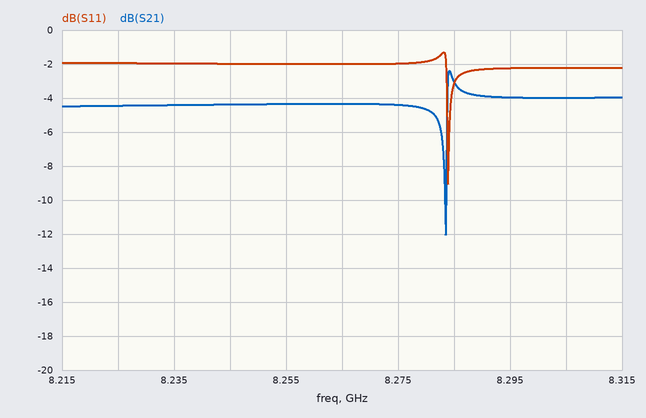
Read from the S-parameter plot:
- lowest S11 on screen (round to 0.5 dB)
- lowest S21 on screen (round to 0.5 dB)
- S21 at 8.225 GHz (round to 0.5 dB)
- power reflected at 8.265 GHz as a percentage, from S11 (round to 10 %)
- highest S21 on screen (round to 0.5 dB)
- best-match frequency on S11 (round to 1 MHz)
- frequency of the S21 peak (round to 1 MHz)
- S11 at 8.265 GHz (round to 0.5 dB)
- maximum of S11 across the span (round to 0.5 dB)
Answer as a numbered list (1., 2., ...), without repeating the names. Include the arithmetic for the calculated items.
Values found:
1. -9.0 dB
2. -12.0 dB
3. -4.5 dB
4. 10^(-2/10) ≈ 63.1 %, so 60 % to the nearest 10 %
5. -2.5 dB
6. 8.284 GHz
7. 8.284 GHz
8. -2.0 dB
9. -1.5 dB
